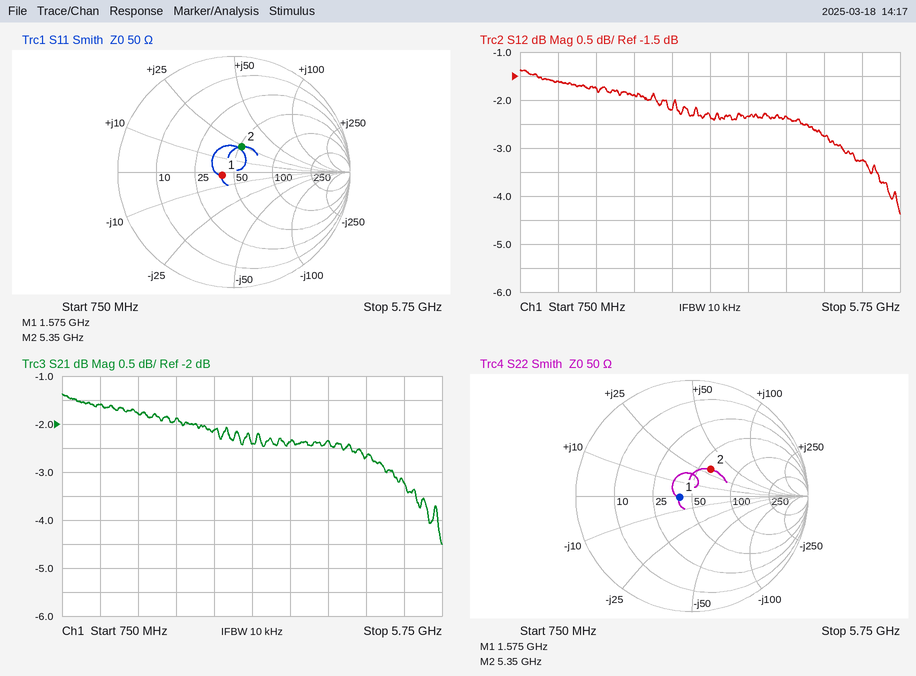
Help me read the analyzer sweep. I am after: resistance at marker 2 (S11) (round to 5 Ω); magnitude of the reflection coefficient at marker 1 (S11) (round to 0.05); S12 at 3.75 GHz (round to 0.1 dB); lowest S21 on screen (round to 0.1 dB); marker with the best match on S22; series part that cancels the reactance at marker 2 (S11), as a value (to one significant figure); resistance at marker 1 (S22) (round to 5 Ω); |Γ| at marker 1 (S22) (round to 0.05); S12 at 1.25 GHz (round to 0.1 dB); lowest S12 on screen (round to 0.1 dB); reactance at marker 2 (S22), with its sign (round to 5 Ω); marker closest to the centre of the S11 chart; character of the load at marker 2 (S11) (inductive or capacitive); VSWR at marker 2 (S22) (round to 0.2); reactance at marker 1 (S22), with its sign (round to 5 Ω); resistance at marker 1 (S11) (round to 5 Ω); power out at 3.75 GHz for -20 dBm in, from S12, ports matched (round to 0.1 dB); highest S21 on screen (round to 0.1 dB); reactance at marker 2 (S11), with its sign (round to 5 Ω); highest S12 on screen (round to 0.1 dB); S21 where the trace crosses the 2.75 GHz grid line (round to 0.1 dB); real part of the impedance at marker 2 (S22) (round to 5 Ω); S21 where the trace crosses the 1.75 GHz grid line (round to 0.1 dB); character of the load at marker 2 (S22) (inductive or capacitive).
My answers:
50 Ω
0.10
-2.3 dB
-4.5 dB
marker 1
1 pF
40 Ω
0.10
-1.6 dB
-4.4 dB
+30 Ω
marker 1
inductive
1.8
0 Ω
40 Ω
-22.3 dBm
-1.4 dB
+25 Ω
-1.4 dB
-2.1 dB
60 Ω
-1.8 dB
inductive
